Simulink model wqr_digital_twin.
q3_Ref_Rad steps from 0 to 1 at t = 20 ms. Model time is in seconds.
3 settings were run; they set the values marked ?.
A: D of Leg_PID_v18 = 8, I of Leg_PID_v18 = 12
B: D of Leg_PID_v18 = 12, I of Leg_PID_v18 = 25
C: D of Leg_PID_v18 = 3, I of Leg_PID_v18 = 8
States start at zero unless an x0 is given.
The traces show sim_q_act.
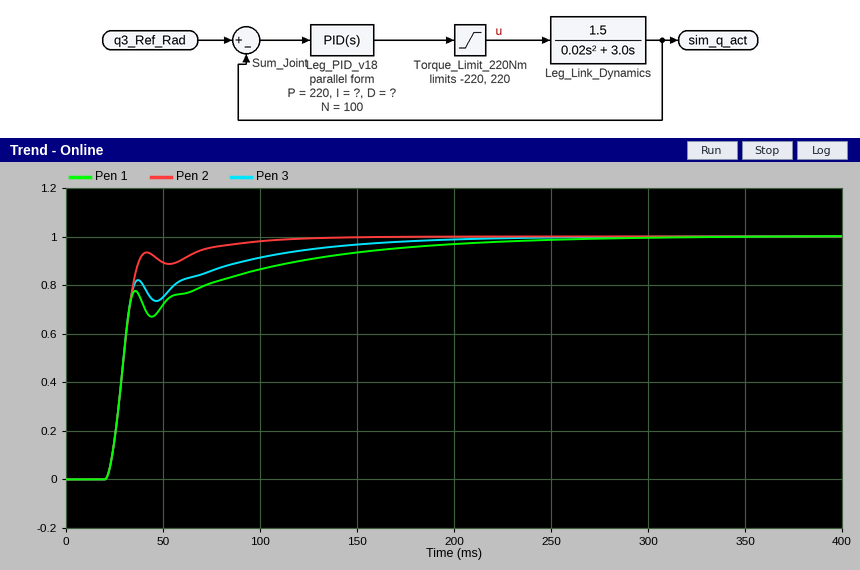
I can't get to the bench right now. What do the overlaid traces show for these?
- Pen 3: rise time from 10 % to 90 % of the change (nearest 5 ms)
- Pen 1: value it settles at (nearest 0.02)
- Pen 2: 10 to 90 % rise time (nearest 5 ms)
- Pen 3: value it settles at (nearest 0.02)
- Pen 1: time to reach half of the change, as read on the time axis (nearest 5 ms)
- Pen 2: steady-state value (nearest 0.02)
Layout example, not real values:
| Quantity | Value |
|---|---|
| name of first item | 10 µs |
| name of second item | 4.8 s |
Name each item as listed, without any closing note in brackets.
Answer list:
| Quantity | Value |
|---|---|
| Pen 3: rise time from 10 % to 90 % of the change | 70 ms |
| Pen 1: value it settles at | 1.00 |
| Pen 2: 10 to 90 % rise time | 15 ms |
| Pen 3: value it settles at | 1.00 |
| Pen 1: time to reach half of the change, as read on the time axis | 30 ms |
| Pen 2: steady-state value | 1.00 |
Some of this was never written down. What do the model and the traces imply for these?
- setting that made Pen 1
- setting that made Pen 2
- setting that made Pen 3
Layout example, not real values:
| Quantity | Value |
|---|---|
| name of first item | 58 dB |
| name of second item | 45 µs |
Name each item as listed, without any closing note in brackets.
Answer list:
| Quantity | Value |
|---|---|
| setting that made Pen 1 | B |
| setting that made Pen 2 | C |
| setting that made Pen 3 | A |
